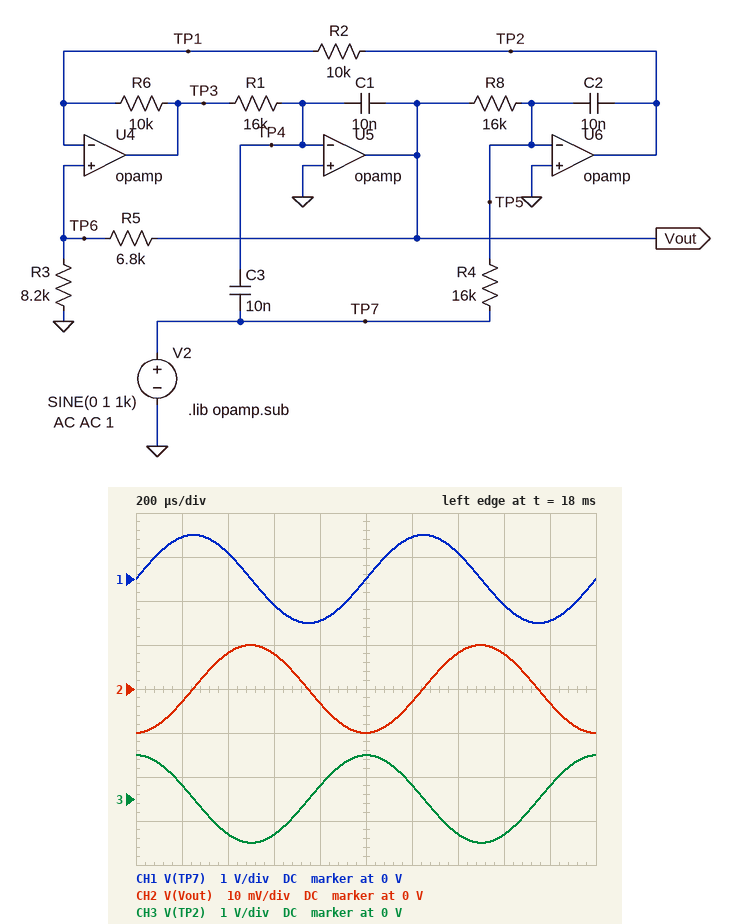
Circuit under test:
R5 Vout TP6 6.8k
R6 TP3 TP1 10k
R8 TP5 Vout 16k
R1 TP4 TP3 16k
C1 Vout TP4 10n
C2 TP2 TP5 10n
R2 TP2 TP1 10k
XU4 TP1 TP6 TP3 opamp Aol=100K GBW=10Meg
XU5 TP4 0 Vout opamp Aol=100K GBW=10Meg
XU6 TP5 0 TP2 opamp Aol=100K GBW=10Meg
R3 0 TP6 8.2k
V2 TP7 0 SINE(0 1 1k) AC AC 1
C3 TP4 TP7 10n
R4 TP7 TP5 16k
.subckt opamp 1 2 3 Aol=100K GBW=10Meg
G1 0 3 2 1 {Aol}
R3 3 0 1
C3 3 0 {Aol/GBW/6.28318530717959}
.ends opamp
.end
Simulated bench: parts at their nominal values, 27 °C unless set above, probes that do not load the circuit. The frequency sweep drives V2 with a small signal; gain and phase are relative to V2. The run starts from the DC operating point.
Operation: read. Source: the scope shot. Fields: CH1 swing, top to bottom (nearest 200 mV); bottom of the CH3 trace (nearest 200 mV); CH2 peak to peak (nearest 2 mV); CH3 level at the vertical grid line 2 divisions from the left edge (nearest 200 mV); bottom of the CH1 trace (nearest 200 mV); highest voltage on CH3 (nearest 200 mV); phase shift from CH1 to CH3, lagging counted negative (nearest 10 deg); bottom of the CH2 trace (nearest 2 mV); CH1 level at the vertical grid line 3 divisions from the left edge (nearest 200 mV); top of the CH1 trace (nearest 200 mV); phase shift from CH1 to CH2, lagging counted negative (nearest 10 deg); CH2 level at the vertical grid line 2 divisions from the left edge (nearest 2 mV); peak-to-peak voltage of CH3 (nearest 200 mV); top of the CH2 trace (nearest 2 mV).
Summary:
2.0 V
-1.0 V
20 mV
-800 mV
-1.0 V
1.0 V
90 deg
-10 mV
-600 mV
1.0 V
-90 deg
8 mV
2.0 V
10 mV
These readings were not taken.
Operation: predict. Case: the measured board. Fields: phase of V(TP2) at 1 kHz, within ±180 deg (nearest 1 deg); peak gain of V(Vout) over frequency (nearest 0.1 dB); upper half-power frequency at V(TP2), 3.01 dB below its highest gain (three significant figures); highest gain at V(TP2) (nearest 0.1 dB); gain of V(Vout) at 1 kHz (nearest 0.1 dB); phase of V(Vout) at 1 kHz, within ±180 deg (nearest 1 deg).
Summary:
89 deg
0 dB
1.14 kHz
1.5 dB
-40.1 dB
-89 deg
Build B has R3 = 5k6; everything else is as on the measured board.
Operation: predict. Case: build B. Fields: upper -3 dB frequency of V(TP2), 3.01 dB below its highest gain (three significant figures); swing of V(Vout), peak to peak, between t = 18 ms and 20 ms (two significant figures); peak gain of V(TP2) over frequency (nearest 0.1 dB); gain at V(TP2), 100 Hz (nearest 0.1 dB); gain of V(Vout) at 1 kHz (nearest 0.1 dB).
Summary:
1.18 kHz
24 mV
1.0 dB
-0.8 dB
-38.4 dB
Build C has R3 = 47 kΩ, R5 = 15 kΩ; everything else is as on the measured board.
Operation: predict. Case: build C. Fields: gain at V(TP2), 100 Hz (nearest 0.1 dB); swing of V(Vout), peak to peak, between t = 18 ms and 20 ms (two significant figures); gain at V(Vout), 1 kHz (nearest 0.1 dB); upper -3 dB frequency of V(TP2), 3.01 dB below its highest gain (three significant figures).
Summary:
3.6 dB
14 mV
-42.9 dB
923 Hz
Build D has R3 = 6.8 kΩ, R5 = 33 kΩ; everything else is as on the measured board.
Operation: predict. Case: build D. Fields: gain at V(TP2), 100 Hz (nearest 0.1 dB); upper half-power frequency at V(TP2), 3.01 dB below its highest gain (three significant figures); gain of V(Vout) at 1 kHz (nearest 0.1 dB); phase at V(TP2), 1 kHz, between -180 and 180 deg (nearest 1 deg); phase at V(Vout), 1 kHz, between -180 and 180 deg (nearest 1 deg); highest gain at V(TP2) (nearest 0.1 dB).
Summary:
-9.2 dB
1.12 kHz
-30.0 dB
88 deg
-90 deg
0.1 dB
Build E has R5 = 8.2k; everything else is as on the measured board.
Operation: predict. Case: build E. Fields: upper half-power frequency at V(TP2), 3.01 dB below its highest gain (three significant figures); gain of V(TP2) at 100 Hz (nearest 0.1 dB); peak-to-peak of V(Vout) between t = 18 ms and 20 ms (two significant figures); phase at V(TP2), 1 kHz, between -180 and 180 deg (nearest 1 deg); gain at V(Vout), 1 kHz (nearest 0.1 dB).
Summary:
1.16 kHz
0 dB
22 mV
89 deg
-39.3 dB
